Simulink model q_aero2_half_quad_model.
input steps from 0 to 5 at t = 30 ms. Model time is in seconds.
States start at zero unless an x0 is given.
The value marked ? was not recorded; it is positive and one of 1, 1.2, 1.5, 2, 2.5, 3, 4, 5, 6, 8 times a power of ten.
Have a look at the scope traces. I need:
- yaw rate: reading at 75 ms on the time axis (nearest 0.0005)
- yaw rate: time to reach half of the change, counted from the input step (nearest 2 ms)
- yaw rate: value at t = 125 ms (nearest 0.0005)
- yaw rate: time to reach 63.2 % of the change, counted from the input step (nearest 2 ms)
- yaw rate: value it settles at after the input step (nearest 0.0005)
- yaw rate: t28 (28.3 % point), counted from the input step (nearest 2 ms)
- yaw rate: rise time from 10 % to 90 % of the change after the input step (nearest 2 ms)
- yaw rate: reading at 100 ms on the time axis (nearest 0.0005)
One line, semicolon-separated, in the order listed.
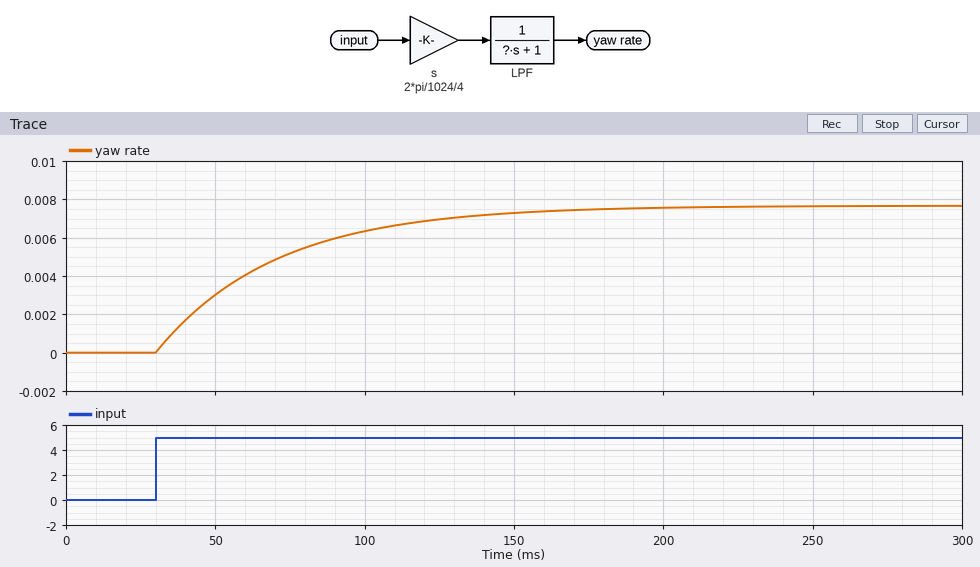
0.0050; 28 ms; 0.0070; 40 ms; 0.0075; 14 ms; 88 ms; 0.0065
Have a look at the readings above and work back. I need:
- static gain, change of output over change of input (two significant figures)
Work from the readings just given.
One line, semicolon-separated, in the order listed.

0.0015
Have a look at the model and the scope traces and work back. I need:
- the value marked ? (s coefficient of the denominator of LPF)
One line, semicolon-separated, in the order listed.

0.04
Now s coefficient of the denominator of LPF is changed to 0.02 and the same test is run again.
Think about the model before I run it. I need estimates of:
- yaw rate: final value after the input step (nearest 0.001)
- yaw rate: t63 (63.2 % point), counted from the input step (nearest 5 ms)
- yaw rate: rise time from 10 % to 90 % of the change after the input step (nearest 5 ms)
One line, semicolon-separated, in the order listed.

0.008; 20 ms; 45 ms
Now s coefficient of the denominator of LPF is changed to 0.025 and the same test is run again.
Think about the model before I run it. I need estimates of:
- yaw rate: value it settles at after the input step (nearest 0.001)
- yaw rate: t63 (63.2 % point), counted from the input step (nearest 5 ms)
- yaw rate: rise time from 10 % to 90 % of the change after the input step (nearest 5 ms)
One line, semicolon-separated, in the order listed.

0.008; 25 ms; 55 ms
